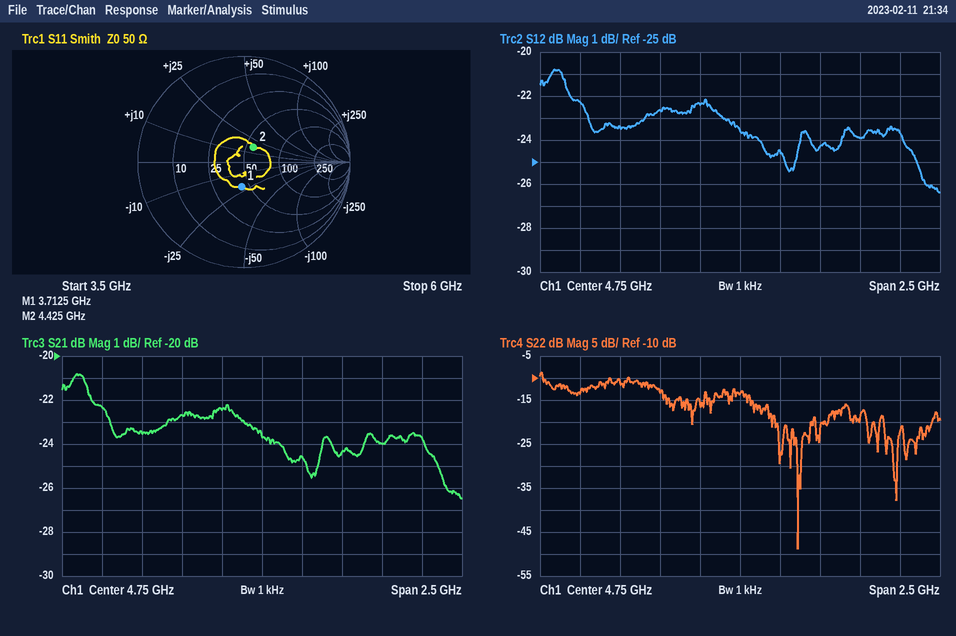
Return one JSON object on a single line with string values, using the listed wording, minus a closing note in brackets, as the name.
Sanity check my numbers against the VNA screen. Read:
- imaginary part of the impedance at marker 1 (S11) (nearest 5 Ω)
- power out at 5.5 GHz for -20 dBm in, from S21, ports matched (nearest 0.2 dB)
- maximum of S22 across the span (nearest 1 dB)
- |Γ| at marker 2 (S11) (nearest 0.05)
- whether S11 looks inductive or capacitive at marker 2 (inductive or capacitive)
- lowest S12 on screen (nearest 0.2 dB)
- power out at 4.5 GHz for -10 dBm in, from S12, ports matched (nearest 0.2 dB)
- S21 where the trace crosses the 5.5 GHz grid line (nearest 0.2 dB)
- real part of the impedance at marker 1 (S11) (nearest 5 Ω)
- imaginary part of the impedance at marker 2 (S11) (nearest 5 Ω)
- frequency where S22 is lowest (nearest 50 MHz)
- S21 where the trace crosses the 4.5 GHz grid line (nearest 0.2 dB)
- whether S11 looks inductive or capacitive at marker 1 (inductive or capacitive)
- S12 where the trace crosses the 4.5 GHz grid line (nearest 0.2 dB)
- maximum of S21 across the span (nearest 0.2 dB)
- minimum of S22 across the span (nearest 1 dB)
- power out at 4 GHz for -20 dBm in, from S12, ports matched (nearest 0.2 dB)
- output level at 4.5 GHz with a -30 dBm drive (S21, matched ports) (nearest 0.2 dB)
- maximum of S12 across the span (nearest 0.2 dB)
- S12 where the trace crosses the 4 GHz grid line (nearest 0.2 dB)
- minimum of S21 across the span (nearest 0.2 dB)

{"imaginary part of the impedance at marker 1 (S11)": "-20 Ω", "power out at 5.5 GHz for -20 dBm in, from S21, ports matched": "-44.0 dBm", "maximum of S22 across the span": "-9 dB", "|Γ| at marker 2 (S11)": "0.15", "whether S11 looks inductive or capacitive at marker 2": "inductive", "lowest S12 on screen": "-26.4 dB", "power out at 4.5 GHz for -10 dBm in, from S12, ports matched": "-32.4 dBm", "S21 where the trace crosses the 5.5 GHz grid line": "-24.0 dB", "real part of the impedance at marker 1 (S11)": "45 Ω", "imaginary part of the impedance at marker 2 (S11)": "+15 Ω", "frequency where S22 is lowest": "5.10 GHz", "S21 where the trace crosses the 4.5 GHz grid line": "-22.4 dB", "whether S11 looks inductive or capacitive at marker 1": "capacitive", "S12 where the trace crosses the 4.5 GHz grid line": "-22.4 dB", "maximum of S21 across the span": "-20.8 dB", "minimum of S22 across the span": "-49 dB", "power out at 4 GHz for -20 dBm in, from S12, ports matched": "-43.4 dBm", "output level at 4.5 GHz with a -30 dBm drive (S21, matched ports)": "-52.4 dBm", "maximum of S12 across the span": "-20.8 dB", "S12 where the trace crosses the 4 GHz grid line": "-23.4 dB", "minimum of S21 across the span": "-26.4 dB"}
